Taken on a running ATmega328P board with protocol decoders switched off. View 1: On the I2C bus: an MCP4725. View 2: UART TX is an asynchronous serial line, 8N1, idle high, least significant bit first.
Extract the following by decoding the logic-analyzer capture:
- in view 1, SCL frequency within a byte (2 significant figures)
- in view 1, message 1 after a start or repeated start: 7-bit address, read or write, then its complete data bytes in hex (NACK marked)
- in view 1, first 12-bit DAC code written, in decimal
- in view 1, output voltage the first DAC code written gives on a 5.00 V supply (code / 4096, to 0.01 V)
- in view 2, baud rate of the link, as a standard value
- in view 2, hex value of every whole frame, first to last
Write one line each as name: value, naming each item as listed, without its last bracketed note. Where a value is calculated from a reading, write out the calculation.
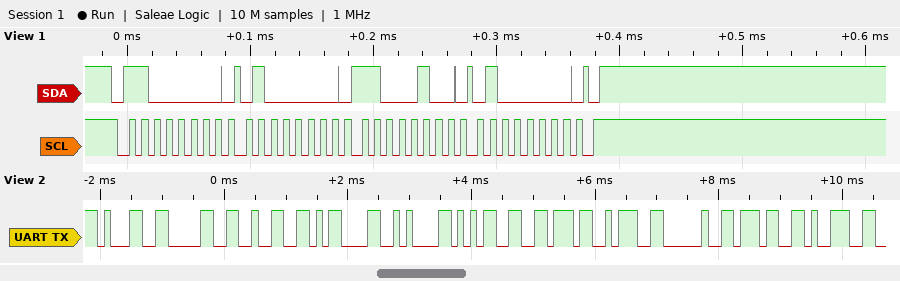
in view 1, SCL frequency within a byte: 100 kHz
in view 1, message 1 after a start or repeated start: 7-bit address, read or write, then its complete data bytes in hex: 0x60 write: 40 C4 40
in view 1, first 12-bit DAC code written, in decimal: 3140
in view 1, output voltage the first DAC code written gives on a 5.00 V supply: 3140 / 4096 x 5.00 V = 3.83 V
in view 2, baud rate of the link, as a standard value: 9600 baud
in view 2, hex value of every whole frame, first to last: 0x31 0x30 0x32 0x0D 0x0A 0x35 0x76 0x3A 0x20 0x37 0x39
